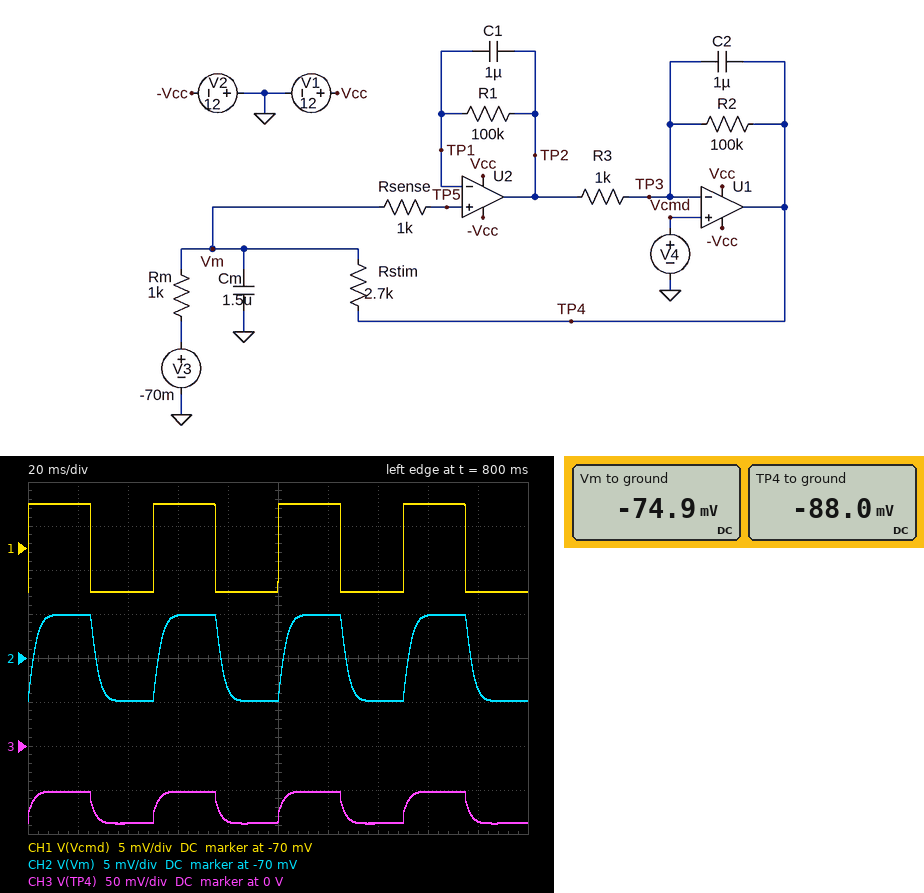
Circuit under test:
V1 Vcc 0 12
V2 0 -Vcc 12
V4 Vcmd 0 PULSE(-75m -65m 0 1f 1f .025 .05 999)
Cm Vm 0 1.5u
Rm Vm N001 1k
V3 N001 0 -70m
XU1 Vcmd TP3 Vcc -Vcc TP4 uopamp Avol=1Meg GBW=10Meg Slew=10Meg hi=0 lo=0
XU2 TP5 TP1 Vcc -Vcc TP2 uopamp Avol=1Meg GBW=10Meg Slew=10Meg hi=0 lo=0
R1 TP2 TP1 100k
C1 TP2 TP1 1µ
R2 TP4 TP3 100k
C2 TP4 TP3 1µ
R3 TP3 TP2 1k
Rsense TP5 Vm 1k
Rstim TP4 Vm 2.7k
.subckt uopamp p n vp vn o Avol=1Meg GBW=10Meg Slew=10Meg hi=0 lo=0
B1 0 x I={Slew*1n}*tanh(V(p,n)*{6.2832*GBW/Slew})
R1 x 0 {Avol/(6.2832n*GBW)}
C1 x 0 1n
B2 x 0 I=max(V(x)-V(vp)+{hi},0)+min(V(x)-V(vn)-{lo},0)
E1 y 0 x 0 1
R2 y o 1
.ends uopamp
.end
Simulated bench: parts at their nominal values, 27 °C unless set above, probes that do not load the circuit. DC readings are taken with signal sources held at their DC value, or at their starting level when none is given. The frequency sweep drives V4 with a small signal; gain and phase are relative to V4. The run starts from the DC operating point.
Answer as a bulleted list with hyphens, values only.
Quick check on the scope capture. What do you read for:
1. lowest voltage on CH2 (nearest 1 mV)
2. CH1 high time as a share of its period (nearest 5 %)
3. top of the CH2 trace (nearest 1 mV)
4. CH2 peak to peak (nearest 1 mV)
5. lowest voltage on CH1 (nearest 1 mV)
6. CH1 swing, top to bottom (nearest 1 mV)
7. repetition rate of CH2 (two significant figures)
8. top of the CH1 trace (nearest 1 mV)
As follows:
- -75 mV
- 50 %
- -65 mV
- 10 mV
- -75 mV
- 10 mV
- 20 Hz
- -65 mV
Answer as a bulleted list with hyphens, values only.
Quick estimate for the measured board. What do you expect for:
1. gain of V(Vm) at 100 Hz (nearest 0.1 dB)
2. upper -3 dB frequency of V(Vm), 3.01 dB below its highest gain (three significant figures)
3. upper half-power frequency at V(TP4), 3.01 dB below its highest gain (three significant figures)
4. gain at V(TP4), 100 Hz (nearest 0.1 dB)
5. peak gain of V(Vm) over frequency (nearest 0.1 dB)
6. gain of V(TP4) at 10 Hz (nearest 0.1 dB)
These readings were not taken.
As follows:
- -6.2 dB
- 65.8 Hz
- 79.2 Hz
- 6.9 dB
- -0.2 dB
- 11.1 dB
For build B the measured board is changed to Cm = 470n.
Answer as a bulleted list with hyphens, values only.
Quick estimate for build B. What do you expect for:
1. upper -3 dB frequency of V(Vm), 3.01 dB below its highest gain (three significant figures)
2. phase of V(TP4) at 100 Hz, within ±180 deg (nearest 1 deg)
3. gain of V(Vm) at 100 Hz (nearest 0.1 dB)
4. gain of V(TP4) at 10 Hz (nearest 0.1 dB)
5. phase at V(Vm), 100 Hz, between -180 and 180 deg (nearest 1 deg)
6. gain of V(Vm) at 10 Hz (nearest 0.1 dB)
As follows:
- 54.3 Hz
- -33 deg
- -6.1 dB
- 11.0 dB
- -45 deg
- -0.4 dB
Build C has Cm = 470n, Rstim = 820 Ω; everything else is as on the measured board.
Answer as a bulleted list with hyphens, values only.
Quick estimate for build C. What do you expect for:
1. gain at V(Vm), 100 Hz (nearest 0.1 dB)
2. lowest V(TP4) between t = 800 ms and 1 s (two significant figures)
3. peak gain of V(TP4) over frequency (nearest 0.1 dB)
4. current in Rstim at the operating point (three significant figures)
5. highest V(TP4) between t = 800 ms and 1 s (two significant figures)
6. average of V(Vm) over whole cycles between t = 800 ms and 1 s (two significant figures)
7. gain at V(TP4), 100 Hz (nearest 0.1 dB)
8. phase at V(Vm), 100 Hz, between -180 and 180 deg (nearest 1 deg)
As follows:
- -1.6 dB
- -79 mV
- 5.1 dB
- 4.96 µA
- -61 mV
- -70 mV
- 3.6 dB
- -21 deg
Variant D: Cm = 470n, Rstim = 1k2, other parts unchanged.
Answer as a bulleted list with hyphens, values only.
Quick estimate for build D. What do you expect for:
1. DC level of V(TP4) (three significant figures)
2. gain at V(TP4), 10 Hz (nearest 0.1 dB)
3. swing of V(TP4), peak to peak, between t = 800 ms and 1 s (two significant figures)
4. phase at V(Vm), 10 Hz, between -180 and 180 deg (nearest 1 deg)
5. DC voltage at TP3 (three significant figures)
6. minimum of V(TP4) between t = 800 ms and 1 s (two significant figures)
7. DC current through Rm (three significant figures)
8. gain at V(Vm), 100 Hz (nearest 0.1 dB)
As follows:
- -80.9 mV
- 6.7 dB
- 22 mV
- -4 deg
- -75.0 mV
- -81 mV
- 4.94 µA
- -2.6 dB
